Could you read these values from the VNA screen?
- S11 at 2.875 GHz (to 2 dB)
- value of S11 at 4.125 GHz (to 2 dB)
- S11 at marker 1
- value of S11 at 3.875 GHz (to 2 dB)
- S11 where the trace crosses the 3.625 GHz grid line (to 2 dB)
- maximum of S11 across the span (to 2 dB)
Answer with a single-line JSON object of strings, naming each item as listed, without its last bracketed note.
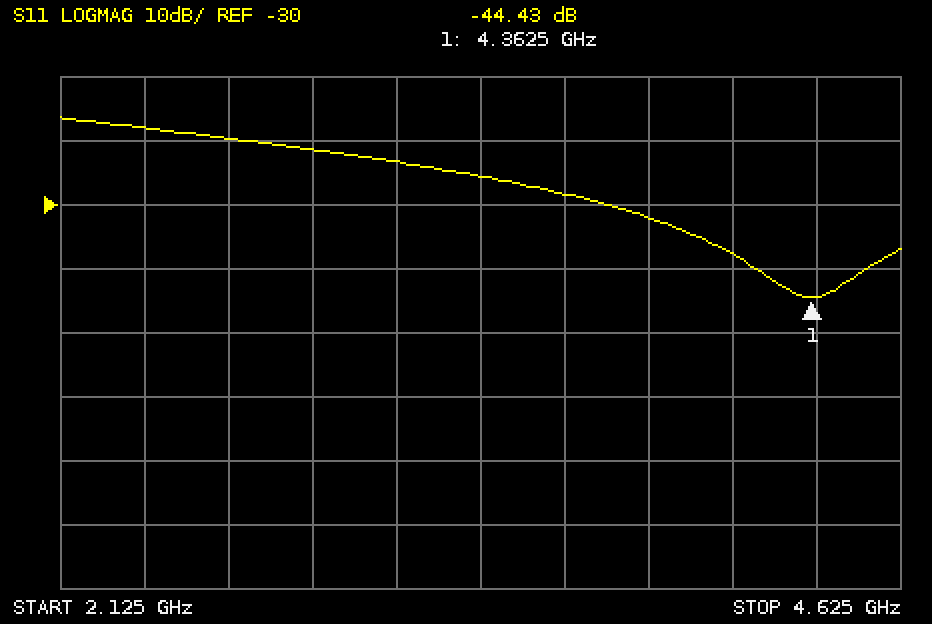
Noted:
{"S11 at 2.875 GHz": "-22 dB", "value of S11 at 4.125 GHz": "-38 dB", "S11 at marker 1": "-44.43 dB", "value of S11 at 3.875 GHz": "-32 dB", "S11 where the trace crosses the 3.625 GHz grid line": "-28 dB", "maximum of S11 across the span": "-16 dB"}
